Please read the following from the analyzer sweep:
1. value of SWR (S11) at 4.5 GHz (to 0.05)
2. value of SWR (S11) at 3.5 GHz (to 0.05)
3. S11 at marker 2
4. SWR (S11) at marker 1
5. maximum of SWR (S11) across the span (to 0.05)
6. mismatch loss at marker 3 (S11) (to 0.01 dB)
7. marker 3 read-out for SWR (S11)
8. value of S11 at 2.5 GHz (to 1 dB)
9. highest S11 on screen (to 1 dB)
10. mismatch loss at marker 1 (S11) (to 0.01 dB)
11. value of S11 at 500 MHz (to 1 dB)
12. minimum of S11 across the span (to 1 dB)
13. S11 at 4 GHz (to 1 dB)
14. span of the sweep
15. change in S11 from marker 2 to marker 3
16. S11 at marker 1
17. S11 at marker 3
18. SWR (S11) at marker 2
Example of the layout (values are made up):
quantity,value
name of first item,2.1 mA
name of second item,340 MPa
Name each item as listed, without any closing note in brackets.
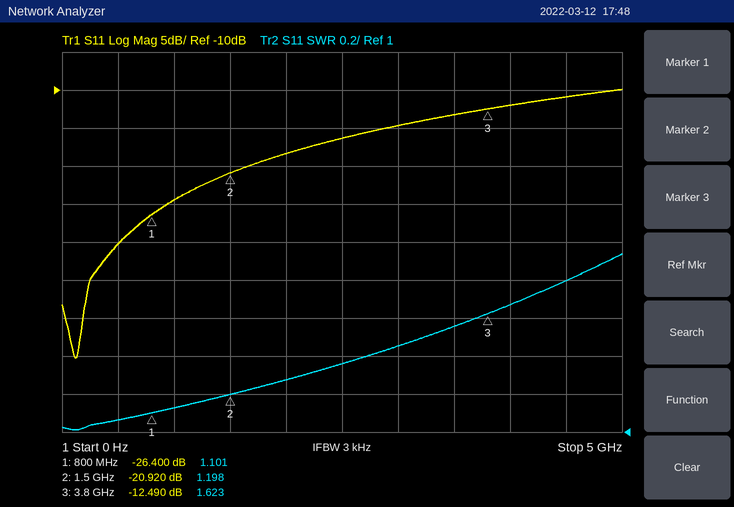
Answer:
quantity,value
value of SWR (S11) at 4.5 GHz,1.80
value of SWR (S11) at 3.5 GHz,1.55
S11 at marker 2,-20.920 dB
SWR (S11) at marker 1,1.101
maximum of SWR (S11) across the span,1.95
mismatch loss at marker 3 (S11),0.25 dB
marker 3 read-out for SWR,1.623
value of S11 at 2.5 GHz,-16 dB
highest S11 on screen,-10 dB
mismatch loss at marker 1 (S11),0.01 dB
value of S11 at 500 MHz,-30 dB
minimum of S11 across the span,-45 dB
S11 at 4 GHz,-12 dB
span of the sweep,5 GHz
change in S11 from marker 2 to marker 3,8.430 dB
S11 at marker 1,-26.400 dB
S11 at marker 3,-12.490 dB
SWR (S11) at marker 2,1.198
